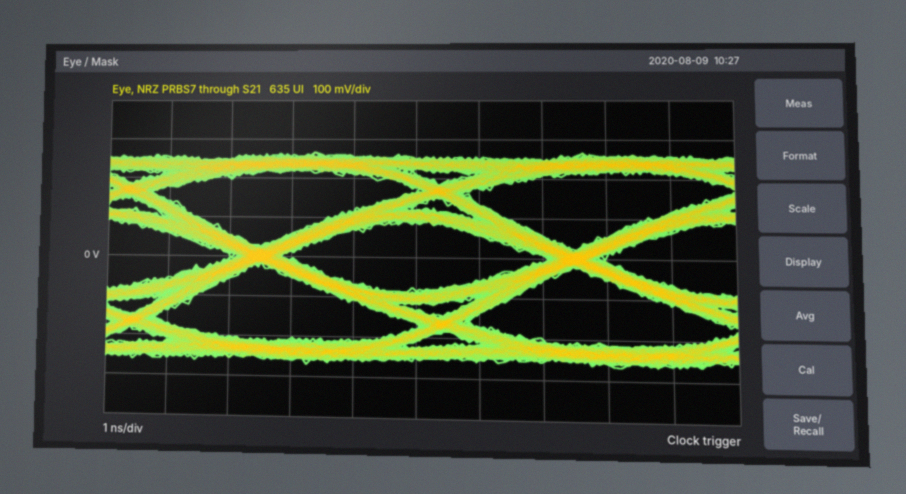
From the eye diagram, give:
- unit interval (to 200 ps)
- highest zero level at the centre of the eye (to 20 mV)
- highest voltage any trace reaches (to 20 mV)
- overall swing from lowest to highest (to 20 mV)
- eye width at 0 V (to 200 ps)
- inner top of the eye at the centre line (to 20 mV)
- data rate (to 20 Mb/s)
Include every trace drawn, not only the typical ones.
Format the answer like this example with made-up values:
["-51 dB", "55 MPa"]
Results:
["5.0 ns", "-80 mV", "260 mV", "540 mV", "4.2 ns", "80 mV", "200 Mb/s"]
